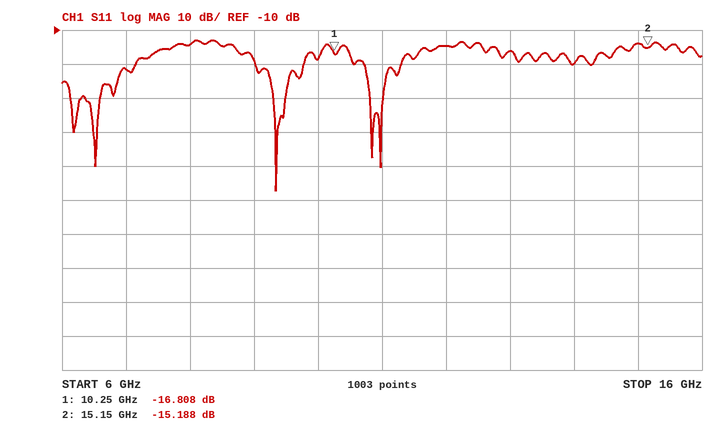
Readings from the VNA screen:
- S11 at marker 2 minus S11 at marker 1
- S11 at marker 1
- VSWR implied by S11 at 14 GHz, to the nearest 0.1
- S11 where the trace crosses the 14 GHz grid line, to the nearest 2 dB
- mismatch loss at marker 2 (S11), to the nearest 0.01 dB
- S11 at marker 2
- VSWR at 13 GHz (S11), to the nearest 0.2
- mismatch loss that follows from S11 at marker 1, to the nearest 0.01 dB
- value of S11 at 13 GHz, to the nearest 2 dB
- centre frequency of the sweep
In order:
1.620 dB
-16.808 dB
1.2
-20 dB
0.13 dB
-15.188 dB
1.4
0.09 dB
-16 dB
11 GHz
